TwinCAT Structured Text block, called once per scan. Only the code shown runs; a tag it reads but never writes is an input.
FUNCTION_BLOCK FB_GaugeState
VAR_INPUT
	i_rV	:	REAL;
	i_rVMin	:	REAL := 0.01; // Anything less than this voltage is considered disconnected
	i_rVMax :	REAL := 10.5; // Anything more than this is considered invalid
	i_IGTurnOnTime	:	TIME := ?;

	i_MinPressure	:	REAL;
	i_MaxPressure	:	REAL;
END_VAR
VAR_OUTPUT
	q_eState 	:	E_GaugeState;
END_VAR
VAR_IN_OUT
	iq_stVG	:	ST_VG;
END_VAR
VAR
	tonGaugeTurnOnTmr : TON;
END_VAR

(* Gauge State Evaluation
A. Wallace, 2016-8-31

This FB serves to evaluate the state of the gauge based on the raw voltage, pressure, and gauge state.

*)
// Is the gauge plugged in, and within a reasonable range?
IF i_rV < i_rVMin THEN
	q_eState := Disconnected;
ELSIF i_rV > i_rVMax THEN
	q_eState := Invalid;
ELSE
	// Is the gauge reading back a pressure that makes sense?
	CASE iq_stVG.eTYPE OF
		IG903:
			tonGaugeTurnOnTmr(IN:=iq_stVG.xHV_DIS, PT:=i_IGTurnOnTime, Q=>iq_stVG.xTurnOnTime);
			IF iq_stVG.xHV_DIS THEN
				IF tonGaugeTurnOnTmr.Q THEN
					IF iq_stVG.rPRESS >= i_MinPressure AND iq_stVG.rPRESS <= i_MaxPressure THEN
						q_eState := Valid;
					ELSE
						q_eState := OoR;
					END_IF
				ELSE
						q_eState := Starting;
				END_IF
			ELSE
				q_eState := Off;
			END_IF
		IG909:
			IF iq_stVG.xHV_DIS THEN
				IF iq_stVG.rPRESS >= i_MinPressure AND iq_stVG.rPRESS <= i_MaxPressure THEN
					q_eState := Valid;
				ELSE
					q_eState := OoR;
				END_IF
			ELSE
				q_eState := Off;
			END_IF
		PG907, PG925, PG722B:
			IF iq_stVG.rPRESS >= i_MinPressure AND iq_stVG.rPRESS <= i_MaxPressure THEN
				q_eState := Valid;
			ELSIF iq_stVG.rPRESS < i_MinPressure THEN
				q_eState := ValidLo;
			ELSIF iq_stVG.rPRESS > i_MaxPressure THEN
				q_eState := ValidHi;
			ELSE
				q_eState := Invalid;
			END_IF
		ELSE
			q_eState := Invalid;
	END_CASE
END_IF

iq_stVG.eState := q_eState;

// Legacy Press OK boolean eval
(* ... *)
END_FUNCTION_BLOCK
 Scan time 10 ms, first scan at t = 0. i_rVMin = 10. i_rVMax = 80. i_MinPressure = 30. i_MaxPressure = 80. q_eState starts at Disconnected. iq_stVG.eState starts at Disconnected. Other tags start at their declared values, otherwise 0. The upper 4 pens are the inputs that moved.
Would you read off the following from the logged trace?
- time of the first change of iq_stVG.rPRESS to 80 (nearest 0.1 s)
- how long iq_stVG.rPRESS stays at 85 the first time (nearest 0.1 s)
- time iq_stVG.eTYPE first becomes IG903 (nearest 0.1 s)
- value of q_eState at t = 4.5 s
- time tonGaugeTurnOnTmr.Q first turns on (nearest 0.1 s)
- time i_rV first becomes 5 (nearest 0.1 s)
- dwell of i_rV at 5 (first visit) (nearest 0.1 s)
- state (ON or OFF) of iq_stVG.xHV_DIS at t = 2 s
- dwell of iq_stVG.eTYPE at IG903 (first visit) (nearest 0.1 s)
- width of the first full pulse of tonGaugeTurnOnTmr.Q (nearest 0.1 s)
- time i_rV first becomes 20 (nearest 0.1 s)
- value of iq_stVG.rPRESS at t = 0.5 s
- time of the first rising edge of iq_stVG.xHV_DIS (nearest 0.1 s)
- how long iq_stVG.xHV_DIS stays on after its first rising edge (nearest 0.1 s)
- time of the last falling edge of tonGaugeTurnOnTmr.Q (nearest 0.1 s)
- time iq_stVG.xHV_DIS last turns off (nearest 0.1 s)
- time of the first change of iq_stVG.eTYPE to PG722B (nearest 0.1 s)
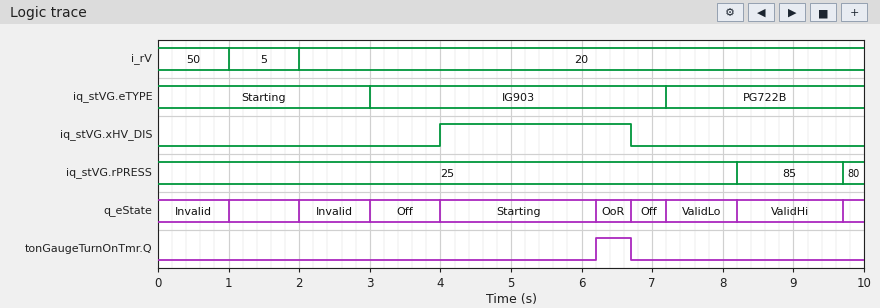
9.7 s
1.5 s
3.0 s
Starting
6.2 s
1.0 s
1.0 s
OFF
4.2 s
0.5 s
2.0 s
25
4.0 s
2.7 s
6.7 s
6.7 s
7.2 s
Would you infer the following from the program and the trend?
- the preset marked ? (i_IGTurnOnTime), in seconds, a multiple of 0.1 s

2.2 s
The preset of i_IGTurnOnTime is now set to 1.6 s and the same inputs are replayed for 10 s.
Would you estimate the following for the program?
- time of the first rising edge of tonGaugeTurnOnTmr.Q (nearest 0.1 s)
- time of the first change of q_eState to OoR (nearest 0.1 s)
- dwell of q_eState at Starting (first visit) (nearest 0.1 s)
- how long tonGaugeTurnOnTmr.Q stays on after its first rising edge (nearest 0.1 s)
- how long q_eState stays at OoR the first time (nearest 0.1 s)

5.6 s
5.6 s
1.6 s
1.1 s
1.1 s
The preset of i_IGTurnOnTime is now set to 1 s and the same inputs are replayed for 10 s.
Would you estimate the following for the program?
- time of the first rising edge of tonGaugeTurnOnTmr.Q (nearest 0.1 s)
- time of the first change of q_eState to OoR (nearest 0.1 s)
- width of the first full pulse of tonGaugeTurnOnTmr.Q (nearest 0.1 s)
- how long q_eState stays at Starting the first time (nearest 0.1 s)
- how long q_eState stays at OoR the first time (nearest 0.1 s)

5.0 s
5.0 s
1.7 s
1.0 s
1.7 s
